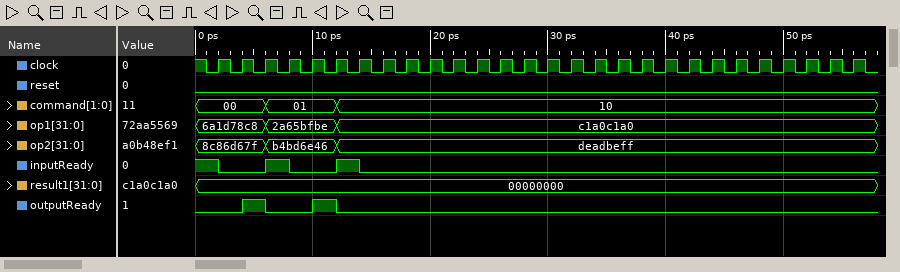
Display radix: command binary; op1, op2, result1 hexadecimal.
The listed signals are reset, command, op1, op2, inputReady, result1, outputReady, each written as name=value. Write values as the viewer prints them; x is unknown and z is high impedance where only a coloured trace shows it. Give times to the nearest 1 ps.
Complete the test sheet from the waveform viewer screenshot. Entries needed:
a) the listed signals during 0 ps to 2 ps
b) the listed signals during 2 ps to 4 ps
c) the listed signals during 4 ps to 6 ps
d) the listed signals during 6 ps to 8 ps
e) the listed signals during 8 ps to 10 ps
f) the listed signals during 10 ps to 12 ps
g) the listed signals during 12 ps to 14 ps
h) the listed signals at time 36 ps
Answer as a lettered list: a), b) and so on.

a) reset=0, command=00, op1=6a1d78c8, op2=8c86d67f, inputReady=1, result1=00000000, outputReady=0
b) reset=0, command=00, op1=6a1d78c8, op2=8c86d67f, inputReady=0, result1=00000000, outputReady=0
c) reset=0, command=00, op1=6a1d78c8, op2=8c86d67f, inputReady=0, result1=00000000, outputReady=1
d) reset=0, command=01, op1=2a65bfbe, op2=b4bd6e46, inputReady=1, result1=00000000, outputReady=0
e) reset=0, command=01, op1=2a65bfbe, op2=b4bd6e46, inputReady=0, result1=00000000, outputReady=0
f) reset=0, command=01, op1=2a65bfbe, op2=b4bd6e46, inputReady=0, result1=00000000, outputReady=1
g) reset=0, command=10, op1=c1a0c1a0, op2=deadbeff, inputReady=1, result1=00000000, outputReady=0
h) reset=0, command=10, op1=c1a0c1a0, op2=deadbeff, inputReady=0, result1=00000000, outputReady=0
